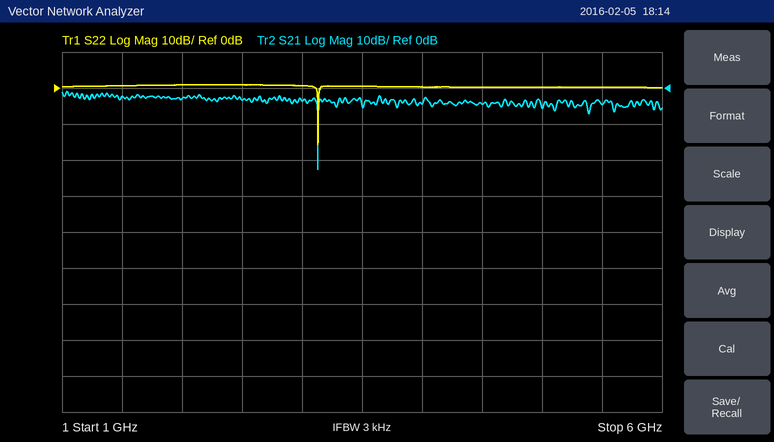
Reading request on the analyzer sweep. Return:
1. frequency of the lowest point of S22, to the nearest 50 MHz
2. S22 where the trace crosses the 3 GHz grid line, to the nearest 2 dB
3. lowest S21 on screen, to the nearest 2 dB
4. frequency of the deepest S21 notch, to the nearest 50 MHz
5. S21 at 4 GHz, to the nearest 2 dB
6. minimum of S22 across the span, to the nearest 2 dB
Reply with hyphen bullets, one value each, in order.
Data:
- 3.15 GHz
- 0 dB
- -22 dB
- 3.15 GHz
- -4 dB
- -16 dB
